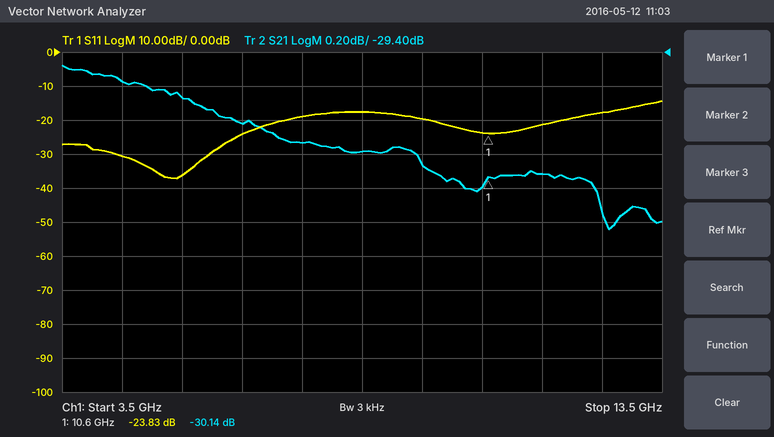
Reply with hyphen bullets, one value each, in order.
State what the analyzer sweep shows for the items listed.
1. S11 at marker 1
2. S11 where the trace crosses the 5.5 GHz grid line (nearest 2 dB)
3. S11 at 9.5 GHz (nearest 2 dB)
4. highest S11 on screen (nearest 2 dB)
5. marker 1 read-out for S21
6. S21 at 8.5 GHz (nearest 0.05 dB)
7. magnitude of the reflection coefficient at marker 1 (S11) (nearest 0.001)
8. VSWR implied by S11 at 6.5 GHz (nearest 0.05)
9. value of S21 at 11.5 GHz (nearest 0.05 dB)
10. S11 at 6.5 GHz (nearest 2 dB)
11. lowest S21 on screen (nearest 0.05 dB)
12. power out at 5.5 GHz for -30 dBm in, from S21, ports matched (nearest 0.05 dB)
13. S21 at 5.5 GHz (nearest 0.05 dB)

- -23.83 dB
- -36 dB
- -20 dB
- -14 dB
- -30.14 dB
- -30.00 dB
- 0.064
- 1.15
- -30.10 dB
- -24 dB
- -30.45 dB
- -59.65 dBm
- -29.65 dB
